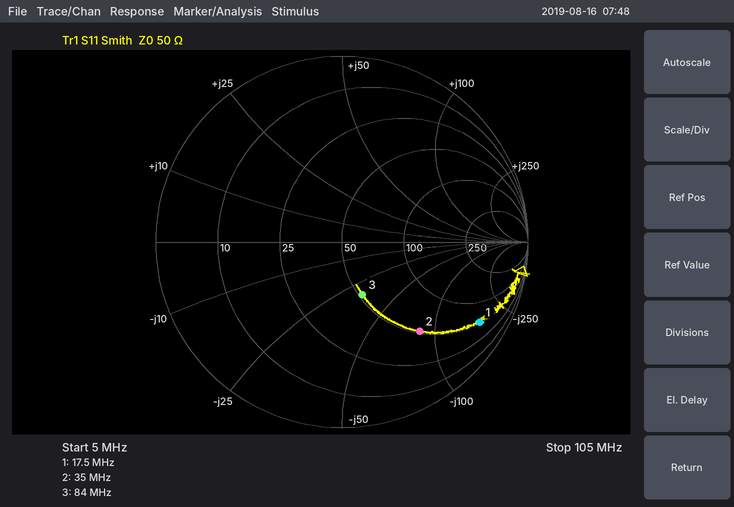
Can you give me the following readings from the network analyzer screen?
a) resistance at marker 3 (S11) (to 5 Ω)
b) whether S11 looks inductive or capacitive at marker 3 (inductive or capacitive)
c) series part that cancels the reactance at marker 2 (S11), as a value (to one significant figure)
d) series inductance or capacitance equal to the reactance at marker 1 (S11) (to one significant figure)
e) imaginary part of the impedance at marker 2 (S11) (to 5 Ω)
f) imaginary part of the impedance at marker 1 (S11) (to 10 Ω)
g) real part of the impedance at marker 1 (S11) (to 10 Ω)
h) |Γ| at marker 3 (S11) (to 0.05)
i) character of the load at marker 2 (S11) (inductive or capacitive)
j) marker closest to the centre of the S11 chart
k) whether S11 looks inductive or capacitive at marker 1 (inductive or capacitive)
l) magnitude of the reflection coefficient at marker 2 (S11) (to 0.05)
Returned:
50 Ω
capacitive
400 nH
50 pF
-85 Ω
-170 Ω
50 Ω
0.30
capacitive
marker 3
capacitive
0.65
